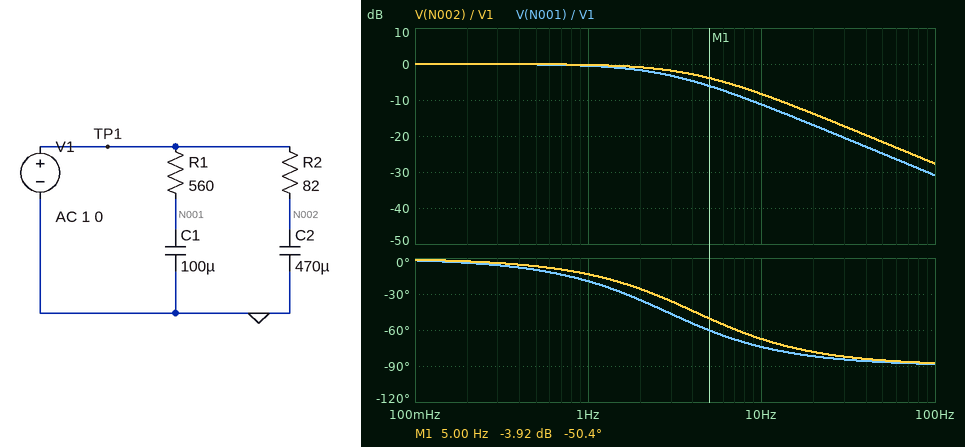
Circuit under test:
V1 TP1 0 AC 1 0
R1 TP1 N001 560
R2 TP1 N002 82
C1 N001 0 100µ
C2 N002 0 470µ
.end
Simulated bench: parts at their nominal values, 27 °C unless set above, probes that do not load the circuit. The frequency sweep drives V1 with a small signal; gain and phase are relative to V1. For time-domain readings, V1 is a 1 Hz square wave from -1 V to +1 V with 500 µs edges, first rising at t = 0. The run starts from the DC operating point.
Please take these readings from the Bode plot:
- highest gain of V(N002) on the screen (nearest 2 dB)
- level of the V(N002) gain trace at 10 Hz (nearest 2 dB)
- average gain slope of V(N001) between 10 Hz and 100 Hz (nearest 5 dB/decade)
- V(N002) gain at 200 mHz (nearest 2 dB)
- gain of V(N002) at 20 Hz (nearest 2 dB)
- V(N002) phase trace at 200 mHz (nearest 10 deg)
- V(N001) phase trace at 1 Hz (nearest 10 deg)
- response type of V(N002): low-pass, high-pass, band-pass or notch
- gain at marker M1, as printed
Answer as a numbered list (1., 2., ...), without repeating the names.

1. 0 dB
2. -8 dB
3. -20 dB/decade
4. 0 dB
5. -14 dB
6. 0 deg
7. -20 deg
8. low-pass
9. -3.92 dB
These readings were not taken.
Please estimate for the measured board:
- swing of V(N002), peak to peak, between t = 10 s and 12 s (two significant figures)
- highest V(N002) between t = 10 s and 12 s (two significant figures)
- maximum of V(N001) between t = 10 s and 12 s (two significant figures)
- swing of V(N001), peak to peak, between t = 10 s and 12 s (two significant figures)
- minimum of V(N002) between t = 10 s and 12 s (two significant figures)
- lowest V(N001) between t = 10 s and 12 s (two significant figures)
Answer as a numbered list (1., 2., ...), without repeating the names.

1. 2.0 V
2. 1.0 V
3. 1.0 V
4. 2.0 V
5. -1.0 V
6. -1.0 V
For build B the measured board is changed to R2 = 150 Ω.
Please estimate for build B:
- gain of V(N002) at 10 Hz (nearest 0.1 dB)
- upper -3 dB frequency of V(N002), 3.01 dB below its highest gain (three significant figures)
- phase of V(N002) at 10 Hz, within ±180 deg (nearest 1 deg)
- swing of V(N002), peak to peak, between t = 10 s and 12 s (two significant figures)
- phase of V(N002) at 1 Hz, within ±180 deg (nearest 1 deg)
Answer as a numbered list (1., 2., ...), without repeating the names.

1. -13.1 dB
2. 2.26 Hz
3. -77 deg
4. 2.0 V
5. -24 deg
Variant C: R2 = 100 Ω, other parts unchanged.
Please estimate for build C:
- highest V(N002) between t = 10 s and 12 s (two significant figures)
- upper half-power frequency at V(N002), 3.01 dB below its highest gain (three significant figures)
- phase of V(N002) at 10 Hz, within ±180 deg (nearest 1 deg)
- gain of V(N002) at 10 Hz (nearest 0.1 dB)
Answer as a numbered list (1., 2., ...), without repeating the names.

1. 1.0 V
2. 3.39 Hz
3. -71 deg
4. -9.9 dB
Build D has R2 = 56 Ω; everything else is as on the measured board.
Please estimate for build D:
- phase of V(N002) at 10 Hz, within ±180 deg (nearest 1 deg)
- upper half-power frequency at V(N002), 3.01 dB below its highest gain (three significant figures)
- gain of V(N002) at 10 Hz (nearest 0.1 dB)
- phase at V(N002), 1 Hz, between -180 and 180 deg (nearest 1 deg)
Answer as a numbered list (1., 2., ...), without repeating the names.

1. -59 deg
2. 6.05 Hz
3. -5.7 dB
4. -9 deg
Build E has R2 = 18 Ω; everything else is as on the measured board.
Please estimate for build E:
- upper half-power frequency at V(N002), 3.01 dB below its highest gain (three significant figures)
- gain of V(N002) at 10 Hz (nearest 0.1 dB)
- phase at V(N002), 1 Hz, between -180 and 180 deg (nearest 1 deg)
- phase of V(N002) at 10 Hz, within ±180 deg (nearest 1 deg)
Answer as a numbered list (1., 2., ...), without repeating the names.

1. 18.8 Hz
2. -1.1 dB
3. -3 deg
4. -28 deg
